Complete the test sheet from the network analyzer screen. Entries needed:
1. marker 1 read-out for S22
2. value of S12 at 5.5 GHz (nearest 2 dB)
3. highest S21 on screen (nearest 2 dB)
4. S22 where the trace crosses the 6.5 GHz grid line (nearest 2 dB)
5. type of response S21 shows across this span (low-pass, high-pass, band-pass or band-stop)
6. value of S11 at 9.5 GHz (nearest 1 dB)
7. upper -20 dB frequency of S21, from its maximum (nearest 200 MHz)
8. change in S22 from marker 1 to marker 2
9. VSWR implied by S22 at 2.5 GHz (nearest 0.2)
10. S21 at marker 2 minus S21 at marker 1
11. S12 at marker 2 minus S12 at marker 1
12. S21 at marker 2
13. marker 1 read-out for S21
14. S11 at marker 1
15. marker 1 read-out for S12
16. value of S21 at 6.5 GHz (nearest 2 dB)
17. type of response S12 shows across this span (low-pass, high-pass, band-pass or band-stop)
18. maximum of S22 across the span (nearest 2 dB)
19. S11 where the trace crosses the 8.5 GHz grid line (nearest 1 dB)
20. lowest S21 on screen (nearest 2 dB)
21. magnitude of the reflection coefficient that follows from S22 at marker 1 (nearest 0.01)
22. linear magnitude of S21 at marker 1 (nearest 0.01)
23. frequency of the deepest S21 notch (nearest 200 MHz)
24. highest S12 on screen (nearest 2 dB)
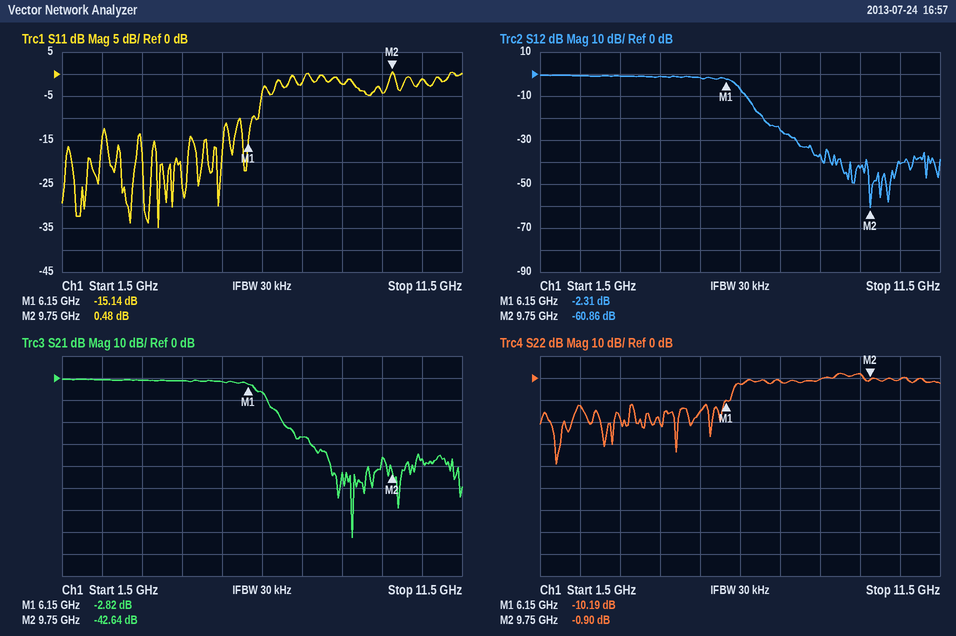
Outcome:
-10.19 dB
-2 dB
0 dB
-2 dB
low-pass
-4 dB
7.0 GHz
9.29 dB
1.6
-39.82 dB
-58.55 dB
-42.64 dB
-2.82 dB
-15.14 dB
-2.31 dB
-6 dB
low-pass
2 dB
-2 dB
-72 dB
0.31
0.72
8.8 GHz
0 dB
